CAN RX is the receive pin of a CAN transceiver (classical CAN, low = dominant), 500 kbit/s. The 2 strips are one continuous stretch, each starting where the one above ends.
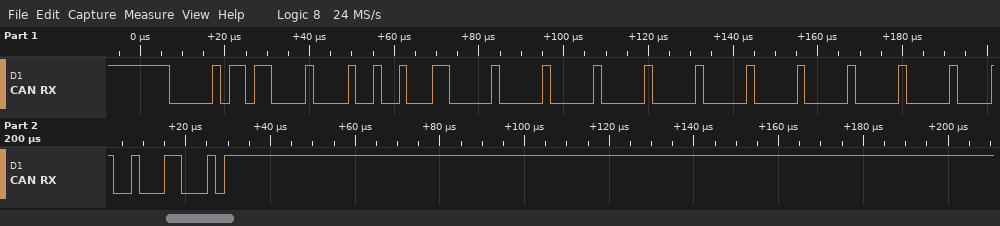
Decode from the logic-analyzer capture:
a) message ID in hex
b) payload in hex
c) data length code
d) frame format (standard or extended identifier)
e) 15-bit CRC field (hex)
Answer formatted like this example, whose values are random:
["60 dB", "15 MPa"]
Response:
["0x036", "49 18 00 00 00 00 00 00", "8", "standard", "0x0918"]
